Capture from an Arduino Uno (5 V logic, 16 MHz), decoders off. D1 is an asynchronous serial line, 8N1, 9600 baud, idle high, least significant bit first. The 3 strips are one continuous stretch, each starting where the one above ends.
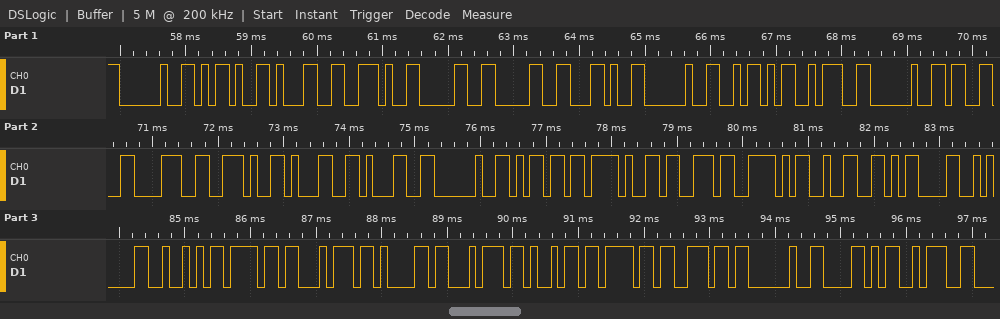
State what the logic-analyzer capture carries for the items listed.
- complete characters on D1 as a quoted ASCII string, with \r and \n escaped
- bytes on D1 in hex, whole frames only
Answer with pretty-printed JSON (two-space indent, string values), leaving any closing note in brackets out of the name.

{
  "complete characters on D1 as a quoted ASCII string, with \\r and \\n escaped": "\" -1.00, Z: 38.11 m/s^2\\r\\nRotation X:\"",
  "bytes on D1 in hex, whole frames only": "20 2D 31 2E 30 30 2C 20 5A 3A 20 33 38 2E 31 31 20 6D 2F 73 5E 32 0D 0A 52 6F 74 61 74 69 6F 6E 20 58 3A"
}
